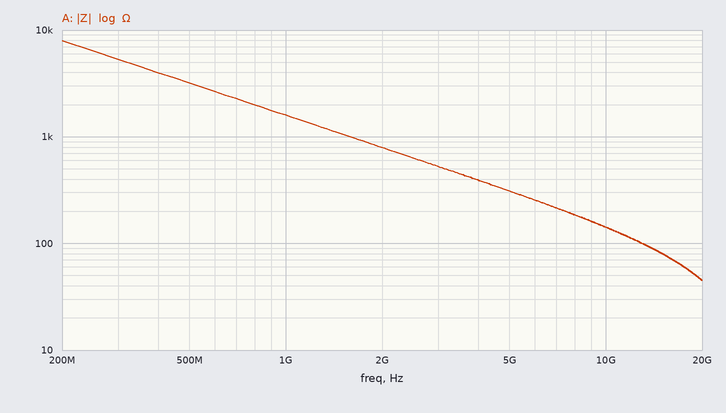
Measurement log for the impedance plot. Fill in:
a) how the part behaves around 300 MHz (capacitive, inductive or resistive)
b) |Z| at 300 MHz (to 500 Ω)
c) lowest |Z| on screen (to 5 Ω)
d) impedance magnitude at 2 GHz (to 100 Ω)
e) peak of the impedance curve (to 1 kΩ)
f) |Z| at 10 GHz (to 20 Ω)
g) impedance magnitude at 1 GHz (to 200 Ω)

capacitive
5.5 kΩ
45 Ω
800 Ω
8 kΩ
140 Ω
1.6 kΩ
